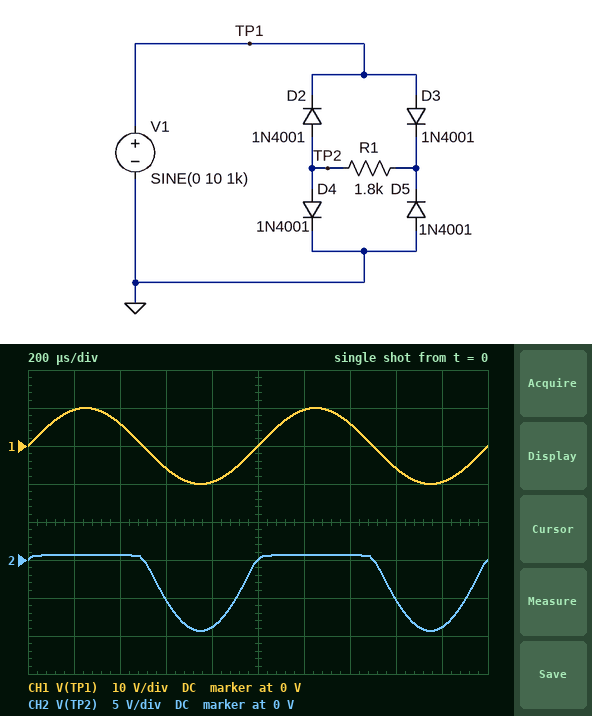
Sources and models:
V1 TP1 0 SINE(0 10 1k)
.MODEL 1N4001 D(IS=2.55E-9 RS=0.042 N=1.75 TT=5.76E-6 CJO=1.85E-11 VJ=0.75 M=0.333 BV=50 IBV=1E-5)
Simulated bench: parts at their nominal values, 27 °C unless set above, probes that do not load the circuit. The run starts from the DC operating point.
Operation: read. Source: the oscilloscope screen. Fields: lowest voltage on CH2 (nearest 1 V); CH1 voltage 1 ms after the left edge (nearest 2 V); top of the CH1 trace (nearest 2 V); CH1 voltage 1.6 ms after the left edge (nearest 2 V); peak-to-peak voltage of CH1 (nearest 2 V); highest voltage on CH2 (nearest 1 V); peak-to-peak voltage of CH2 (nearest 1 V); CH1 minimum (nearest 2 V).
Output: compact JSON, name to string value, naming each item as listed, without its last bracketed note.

{"lowest voltage on CH2": "-9 V", "CH1 voltage 1 ms after the left edge": "0 V", "top of the CH1 trace": "10 V", "CH1 voltage 1.6 ms after the left edge": "-6 V", "peak-to-peak voltage of CH1": "20 V", "highest voltage on CH2": "1 V", "peak-to-peak voltage of CH2": "10 V", "CH1 minimum": "-10 V"}
